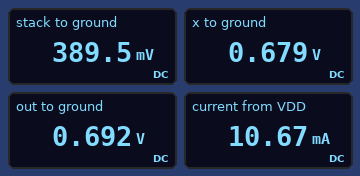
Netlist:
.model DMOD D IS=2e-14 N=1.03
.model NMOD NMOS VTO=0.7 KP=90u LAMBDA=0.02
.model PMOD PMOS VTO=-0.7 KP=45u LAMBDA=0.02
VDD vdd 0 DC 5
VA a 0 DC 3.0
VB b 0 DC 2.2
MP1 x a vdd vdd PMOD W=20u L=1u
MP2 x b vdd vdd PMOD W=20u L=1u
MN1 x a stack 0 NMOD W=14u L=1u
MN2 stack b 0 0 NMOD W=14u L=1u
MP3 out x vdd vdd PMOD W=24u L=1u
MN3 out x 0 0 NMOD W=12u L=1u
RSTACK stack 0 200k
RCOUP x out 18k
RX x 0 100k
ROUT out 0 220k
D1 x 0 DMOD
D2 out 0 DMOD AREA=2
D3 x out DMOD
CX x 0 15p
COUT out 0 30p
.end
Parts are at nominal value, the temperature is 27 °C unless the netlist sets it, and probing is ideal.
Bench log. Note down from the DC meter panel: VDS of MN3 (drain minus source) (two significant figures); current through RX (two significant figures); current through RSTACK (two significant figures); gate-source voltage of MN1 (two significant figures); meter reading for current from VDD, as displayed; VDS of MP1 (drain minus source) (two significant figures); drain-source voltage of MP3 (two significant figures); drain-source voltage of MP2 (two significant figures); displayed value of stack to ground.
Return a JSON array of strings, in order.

["690 mV", "6.8 µA", "1.9 µA", "2.6 V", "10.67 mA", "-4.3 V", "-4.3 V", "-4.3 V", "389.5 mV"]
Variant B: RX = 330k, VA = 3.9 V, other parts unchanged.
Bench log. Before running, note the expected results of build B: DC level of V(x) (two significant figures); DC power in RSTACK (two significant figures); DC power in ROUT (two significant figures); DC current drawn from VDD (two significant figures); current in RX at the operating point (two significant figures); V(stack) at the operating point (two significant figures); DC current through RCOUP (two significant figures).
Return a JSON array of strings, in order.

["670 mV", "1.0 µW", "2.2 µW", "10 mA", "2.0 µA", "450 mV", "1.4 µA"]
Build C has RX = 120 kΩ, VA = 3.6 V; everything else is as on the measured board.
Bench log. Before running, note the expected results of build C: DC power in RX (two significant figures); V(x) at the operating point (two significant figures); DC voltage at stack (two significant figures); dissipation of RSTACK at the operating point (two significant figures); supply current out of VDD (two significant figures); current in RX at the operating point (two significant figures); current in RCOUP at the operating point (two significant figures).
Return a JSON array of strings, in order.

["3.7 µW", "670 mV", "430 mV", "930 nW", "10 mA", "5.6 µA", "1.2 µA"]
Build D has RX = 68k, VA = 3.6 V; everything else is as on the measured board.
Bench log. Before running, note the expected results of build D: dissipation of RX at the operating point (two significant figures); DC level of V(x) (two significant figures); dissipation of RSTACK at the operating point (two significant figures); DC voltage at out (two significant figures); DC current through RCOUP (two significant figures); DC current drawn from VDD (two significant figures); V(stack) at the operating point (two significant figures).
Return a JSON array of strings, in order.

["6.6 µW", "670 mV", "930 nW", "690 mV", "1.2 µA", "10 mA", "430 mV"]
